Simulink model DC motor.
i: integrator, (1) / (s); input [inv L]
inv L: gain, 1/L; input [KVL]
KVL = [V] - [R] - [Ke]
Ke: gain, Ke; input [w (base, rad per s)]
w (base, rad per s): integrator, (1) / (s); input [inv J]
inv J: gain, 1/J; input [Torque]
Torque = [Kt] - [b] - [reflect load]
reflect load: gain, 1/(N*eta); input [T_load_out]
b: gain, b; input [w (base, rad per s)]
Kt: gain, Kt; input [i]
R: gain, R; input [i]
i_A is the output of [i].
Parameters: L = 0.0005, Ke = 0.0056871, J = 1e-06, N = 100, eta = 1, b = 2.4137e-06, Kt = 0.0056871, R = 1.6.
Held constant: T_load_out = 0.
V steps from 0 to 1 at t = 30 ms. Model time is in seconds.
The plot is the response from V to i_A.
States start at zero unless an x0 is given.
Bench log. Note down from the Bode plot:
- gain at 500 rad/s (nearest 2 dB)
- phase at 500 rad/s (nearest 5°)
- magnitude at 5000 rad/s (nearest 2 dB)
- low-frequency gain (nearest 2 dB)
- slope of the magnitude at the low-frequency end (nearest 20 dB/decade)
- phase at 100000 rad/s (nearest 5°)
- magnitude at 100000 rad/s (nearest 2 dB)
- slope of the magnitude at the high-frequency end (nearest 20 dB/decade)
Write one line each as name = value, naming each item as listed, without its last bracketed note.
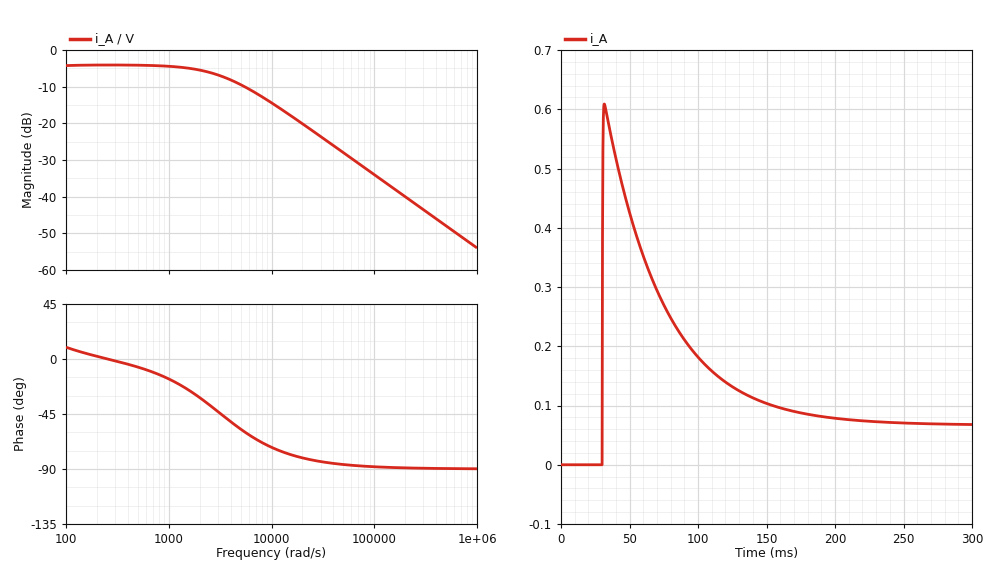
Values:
gain at 500 rad/s = -4 dB
phase at 500 rad/s = -5°
magnitude at 5000 rad/s = -10 dB
low-frequency gain = -4 dB
slope of the magnitude at the low-frequency end = 0 dB/decade
phase at 100000 rad/s = -90°
magnitude at 100000 rad/s = -34 dB
slope of the magnitude at the high-frequency end = -20 dB/decade
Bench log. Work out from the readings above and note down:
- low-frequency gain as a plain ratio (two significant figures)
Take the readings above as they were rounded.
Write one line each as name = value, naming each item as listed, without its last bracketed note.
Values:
low-frequency gain as a plain ratio = 0.63
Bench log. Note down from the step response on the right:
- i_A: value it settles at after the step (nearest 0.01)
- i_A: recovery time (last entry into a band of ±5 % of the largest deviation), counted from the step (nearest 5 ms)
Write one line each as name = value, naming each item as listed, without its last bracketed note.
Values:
i_A: value it settles at after the step = 0.07
i_A: recovery time (last entry into a band of ±5 % of the largest deviation), counted from the step = 130 ms
